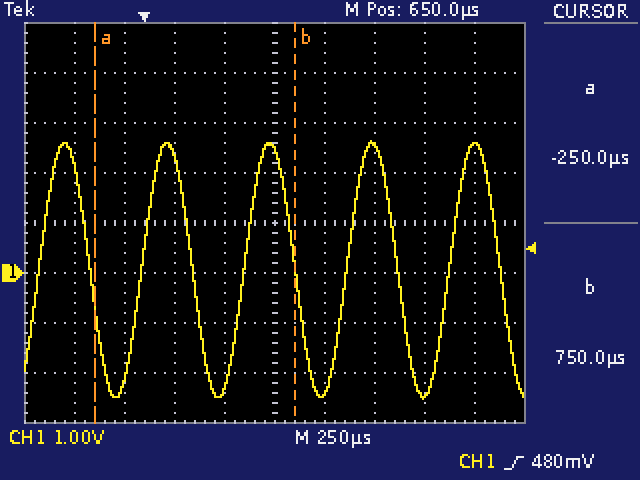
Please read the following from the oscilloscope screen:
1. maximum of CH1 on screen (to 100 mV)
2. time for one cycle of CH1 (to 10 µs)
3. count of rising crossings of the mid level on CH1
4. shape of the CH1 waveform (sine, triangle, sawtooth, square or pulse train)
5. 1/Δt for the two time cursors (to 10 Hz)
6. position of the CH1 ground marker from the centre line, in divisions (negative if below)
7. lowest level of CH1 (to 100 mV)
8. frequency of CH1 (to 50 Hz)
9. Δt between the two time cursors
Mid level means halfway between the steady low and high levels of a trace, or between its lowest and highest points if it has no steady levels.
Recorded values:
2.6 V
510 µs
5
sine
1.00 kHz
-1.0 div
-2.5 V
1.95 kHz
1.000 ms
